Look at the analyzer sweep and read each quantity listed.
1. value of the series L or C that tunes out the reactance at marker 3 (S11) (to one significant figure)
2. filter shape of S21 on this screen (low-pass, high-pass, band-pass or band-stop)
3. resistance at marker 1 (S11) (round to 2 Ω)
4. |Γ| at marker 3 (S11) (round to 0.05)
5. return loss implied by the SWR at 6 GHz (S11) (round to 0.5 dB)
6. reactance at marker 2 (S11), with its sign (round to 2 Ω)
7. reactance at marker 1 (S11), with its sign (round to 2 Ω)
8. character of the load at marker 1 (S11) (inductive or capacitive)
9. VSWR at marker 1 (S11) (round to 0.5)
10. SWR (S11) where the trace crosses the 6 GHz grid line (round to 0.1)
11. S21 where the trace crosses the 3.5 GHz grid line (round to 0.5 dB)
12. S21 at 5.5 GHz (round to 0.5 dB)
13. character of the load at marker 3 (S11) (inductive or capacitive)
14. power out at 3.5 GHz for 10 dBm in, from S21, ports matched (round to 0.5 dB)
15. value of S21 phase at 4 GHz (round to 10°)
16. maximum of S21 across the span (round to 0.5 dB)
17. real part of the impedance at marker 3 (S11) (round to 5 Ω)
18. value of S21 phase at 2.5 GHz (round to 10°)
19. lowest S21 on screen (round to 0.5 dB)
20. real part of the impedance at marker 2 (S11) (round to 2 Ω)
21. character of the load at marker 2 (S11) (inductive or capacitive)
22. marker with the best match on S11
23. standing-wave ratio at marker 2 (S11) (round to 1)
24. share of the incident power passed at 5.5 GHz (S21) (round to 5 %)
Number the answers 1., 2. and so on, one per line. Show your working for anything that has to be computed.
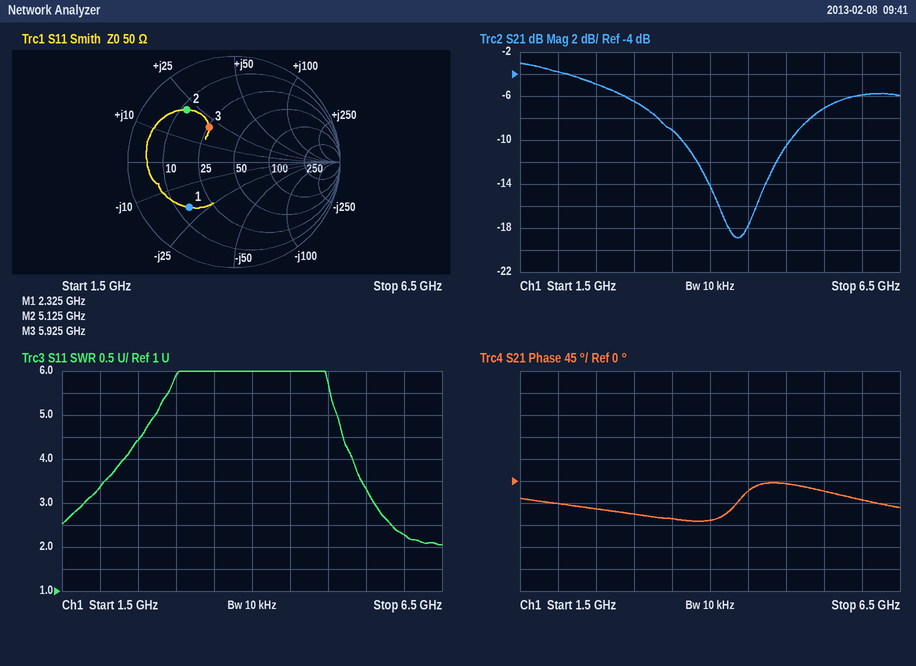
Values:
1. C = 1/(2π × 5.925 GHz × 20 Ω) ≈ 1 pF
2. band-stop
3. 14 Ω
4. 0.40
5. −20 log10((2.3 − 1)/(2.3 + 1)) ≈ 8.09 dB, so 8.0 dB to the nearest 0.5 dB
6. +22 Ω
7. -20 Ω
8. capacitive
9. 4.0
10. 2.3
11. -9.0 dB
12. -7.0 dB
13. inductive
14. 10 dBm + (-9.0 dB) = 1.0 dBm
15. -80°
16. -3.0 dB
17. 25 Ω
18. -60°
19. -19.0 dB
20. 12 Ω
21. inductive
22. marker 3
23. 5
24. 10^(-7/10) ≈ 20 %
